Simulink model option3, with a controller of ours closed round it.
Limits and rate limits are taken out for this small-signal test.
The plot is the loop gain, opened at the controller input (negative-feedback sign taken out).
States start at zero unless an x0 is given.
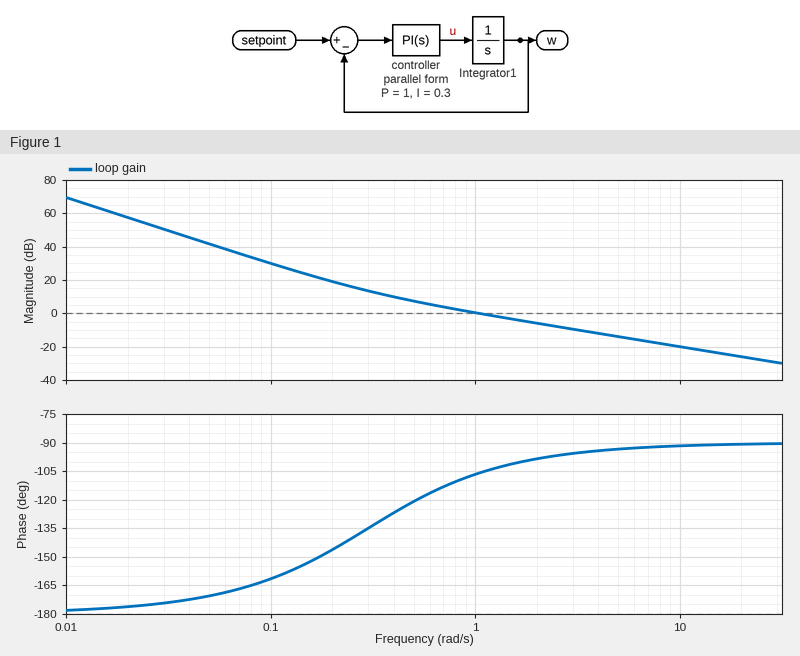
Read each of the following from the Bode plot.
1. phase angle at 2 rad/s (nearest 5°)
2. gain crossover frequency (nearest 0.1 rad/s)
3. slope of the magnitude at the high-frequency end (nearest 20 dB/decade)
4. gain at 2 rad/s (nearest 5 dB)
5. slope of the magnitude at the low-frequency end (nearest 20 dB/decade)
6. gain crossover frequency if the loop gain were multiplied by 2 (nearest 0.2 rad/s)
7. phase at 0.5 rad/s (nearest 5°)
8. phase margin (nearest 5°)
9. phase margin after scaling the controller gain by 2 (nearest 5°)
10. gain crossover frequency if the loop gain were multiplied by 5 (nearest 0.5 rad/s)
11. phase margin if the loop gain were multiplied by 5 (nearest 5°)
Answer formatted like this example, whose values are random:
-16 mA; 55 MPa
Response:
-100°; 1.0 rad/s; -20 dB/decade; -5 dB; -40 dB/decade; 2.0 rad/s; -120°; 75°; 80°; 5.0 rad/s; 85°
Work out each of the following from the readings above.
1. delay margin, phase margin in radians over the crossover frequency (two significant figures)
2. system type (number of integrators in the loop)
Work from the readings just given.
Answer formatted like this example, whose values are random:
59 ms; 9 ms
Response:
1.3 s; 2
